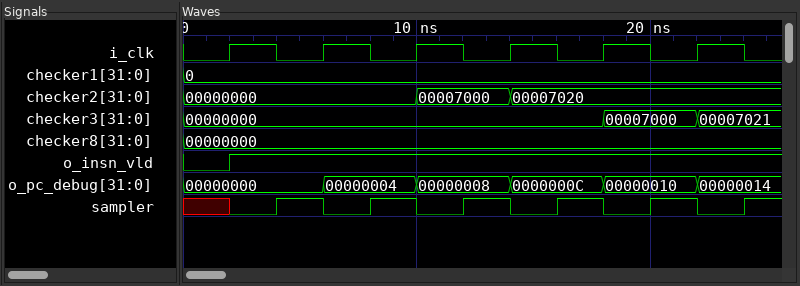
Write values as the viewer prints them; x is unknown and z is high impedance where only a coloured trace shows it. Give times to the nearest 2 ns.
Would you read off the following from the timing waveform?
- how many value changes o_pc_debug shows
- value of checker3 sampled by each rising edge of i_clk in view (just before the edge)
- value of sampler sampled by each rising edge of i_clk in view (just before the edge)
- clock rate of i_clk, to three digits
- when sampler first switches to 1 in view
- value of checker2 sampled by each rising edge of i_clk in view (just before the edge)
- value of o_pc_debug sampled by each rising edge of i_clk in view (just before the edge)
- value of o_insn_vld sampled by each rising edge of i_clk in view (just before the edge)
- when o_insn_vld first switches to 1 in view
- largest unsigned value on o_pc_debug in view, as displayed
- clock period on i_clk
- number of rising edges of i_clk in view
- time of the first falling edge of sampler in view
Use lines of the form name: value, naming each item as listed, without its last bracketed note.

how many value changes o_pc_debug shows: 5
value of checker3 sampled by each rising edge of i_clk in view: 00000000, 00000000, 00000000, 00000000, 00000000, 00007000
value of sampler sampled by each rising edge of i_clk in view: x 1 1 1 1 1
clock rate of i_clk, to three digits: 250 MHz
when sampler first switches to 1 in view: 4 ns
value of checker2 sampled by each rising edge of i_clk in view: 00000000, 00000000, 00000000, 00007000, 00007020, 00007020
value of o_pc_debug sampled by each rising edge of i_clk in view: 00000000, 00000000, 00000004, 00000008, 0000000C, 00000010
value of o_insn_vld sampled by each rising edge of i_clk in view: 0 1 1 1 1 1
when o_insn_vld first switches to 1 in view: 2 ns
largest unsigned value on o_pc_debug in view, as displayed: 00000014
clock period on i_clk: 4 ns
number of rising edges of i_clk in view: 6
time of the first falling edge of sampler in view: 6 ns
